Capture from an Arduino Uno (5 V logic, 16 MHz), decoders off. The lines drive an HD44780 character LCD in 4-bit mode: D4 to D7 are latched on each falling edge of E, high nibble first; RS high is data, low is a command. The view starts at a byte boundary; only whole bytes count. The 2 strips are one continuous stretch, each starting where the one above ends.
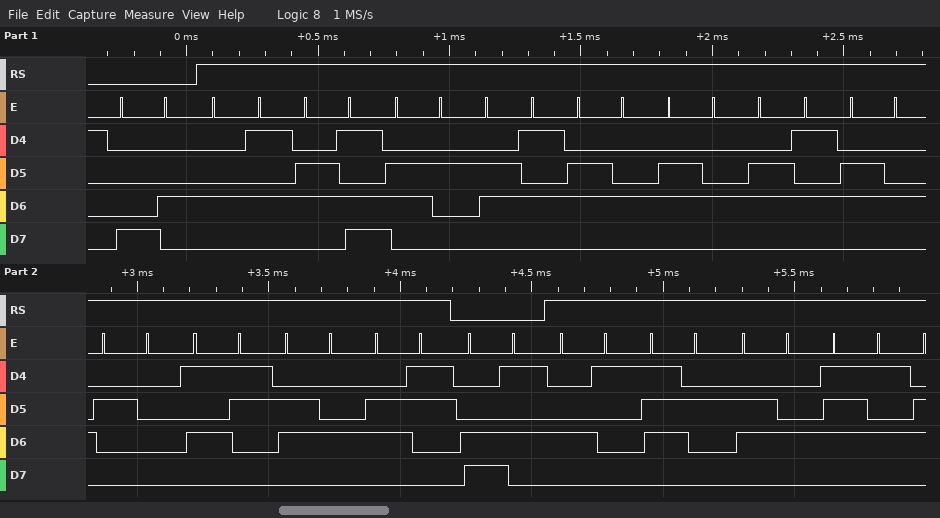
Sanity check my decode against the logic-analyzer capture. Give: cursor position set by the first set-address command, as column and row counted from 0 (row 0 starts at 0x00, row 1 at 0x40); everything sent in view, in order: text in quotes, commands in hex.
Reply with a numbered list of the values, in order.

1. column 4, row 0
2. 0x84 "Embedded Sdc" 0xC5 "Ardu"
